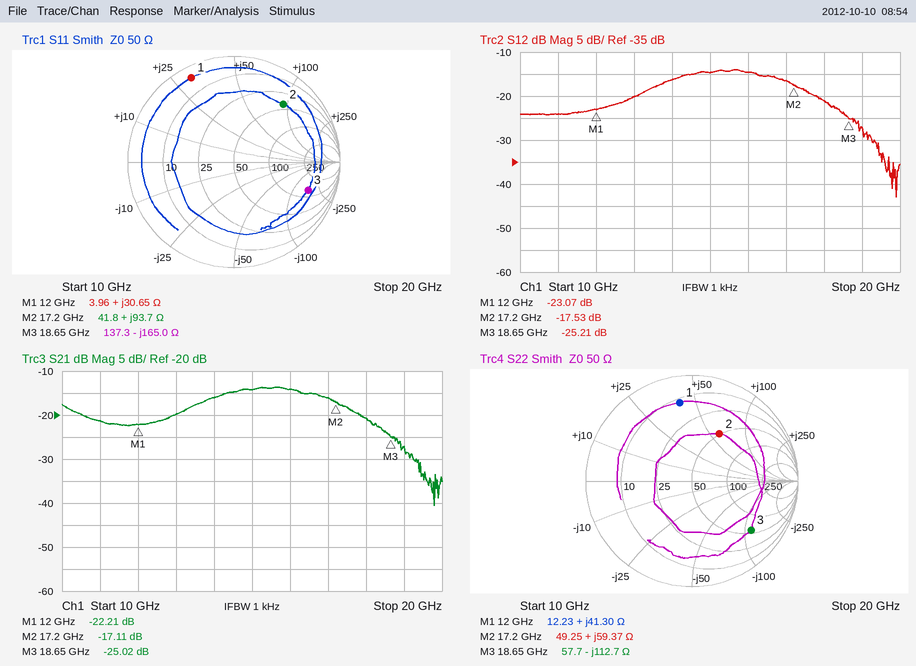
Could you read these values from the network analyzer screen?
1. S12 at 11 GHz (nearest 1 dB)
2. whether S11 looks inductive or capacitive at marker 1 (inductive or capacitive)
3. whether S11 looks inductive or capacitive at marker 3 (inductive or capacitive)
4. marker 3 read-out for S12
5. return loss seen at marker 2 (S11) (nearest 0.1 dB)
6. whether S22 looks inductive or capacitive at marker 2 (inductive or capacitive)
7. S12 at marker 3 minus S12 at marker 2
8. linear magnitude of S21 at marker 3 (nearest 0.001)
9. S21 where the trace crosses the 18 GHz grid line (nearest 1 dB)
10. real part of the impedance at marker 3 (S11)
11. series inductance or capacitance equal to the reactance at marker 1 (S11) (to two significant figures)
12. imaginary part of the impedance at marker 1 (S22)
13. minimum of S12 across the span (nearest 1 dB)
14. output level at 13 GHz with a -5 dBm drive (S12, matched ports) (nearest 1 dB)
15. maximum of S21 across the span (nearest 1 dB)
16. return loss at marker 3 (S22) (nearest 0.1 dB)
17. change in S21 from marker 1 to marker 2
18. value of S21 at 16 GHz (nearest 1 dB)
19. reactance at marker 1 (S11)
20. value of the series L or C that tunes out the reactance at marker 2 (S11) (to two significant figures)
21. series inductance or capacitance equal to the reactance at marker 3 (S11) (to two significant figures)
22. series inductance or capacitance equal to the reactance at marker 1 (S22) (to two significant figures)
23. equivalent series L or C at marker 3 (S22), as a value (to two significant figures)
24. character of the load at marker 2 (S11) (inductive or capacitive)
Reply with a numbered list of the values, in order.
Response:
1. -24 dB
2. inductive
3. capacitive
4. -25.21 dB
5. 2.9 dB
6. inductive
7. -7.68 dB
8. 0.056
9. -21 dB
10. 137.3 Ω
11. 410 pH
12. +41.30 Ω
13. -43 dB
14. -25 dBm
15. -14 dB
16. 2.8 dB
17. 5.10 dB
18. -14 dB
19. +30.65 Ω
20. 99 fF
21. 52 fF
22. 550 pH
23. 76 fF
24. inductive
